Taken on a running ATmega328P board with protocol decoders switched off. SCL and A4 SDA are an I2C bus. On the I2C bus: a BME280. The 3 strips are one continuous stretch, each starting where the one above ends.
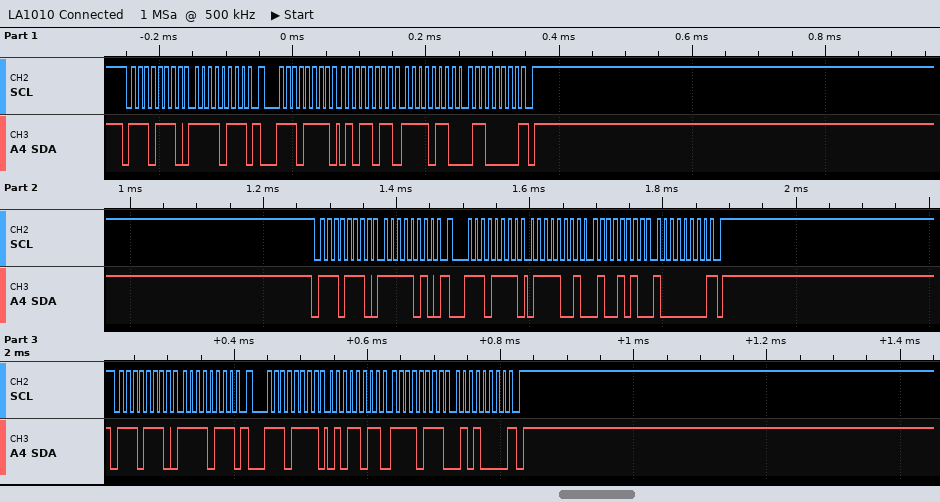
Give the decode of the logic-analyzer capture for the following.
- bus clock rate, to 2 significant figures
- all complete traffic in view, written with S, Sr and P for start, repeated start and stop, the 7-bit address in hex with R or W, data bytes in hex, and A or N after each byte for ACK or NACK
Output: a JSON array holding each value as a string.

["100 kHz", "S 77W A F7 A Sr 77R A 5B A F6 A 60 N P S 77W A FA A Sr 77R A 79 A 4A A 80 N P S 77W A F7 A Sr 77R A 5B A F7 A 50 N P"]
